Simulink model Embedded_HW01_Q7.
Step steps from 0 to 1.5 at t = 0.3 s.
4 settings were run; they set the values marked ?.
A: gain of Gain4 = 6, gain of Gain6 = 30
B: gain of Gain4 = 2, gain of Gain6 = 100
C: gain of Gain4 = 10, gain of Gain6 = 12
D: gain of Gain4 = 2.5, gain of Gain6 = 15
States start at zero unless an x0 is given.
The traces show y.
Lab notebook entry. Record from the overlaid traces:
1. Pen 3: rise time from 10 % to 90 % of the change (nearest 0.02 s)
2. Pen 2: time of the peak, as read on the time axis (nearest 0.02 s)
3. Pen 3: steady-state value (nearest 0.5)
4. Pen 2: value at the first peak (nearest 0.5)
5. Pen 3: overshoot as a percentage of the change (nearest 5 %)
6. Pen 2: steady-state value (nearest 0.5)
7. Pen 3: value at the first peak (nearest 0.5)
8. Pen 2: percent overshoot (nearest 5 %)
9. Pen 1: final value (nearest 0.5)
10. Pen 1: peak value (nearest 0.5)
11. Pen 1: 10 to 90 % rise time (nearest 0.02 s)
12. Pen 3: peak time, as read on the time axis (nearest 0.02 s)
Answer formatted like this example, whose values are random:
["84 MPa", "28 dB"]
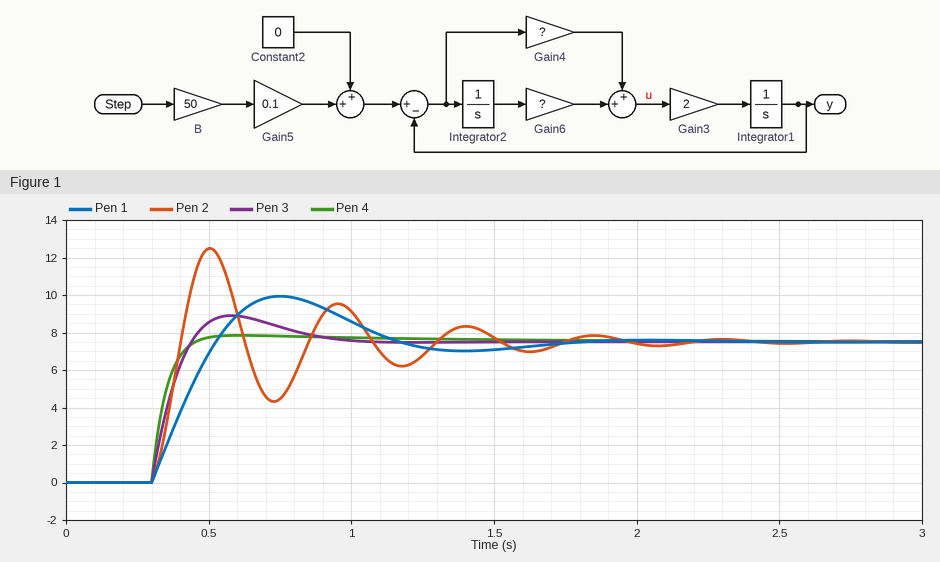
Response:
["0.10 s", "0.50 s", "7.5", "12.5", "20 %", "7.5", "9.0", "65 %", "7.5", "10.0", "0.18 s", "0.58 s"]
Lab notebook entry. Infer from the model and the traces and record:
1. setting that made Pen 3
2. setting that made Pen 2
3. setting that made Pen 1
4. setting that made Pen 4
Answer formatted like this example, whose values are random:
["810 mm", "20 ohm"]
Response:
["A", "B", "D", "C"]
